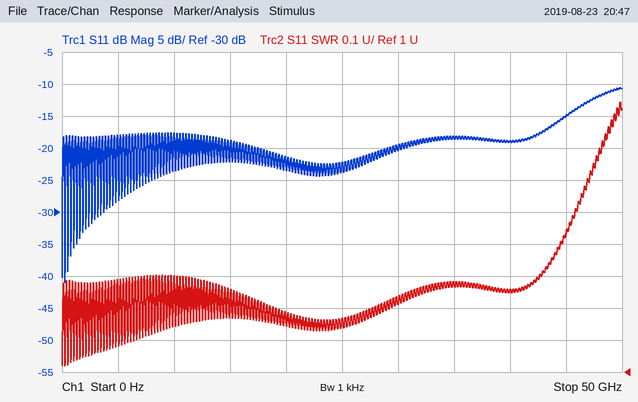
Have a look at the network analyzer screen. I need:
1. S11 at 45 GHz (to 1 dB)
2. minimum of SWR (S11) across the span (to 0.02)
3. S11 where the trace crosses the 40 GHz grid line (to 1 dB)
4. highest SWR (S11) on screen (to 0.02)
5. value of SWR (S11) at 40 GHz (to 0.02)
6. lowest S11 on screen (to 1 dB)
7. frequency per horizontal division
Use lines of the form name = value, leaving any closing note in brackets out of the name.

S11 at 45 GHz = -15 dB
minimum of SWR (S11) across the span = 1.02
S11 where the trace crosses the 40 GHz grid line = -19 dB
highest SWR (S11) on screen = 1.84
value of SWR (S11) at 40 GHz = 1.26
lowest S11 on screen = -41 dB
frequency per horizontal division = 5 GHz
